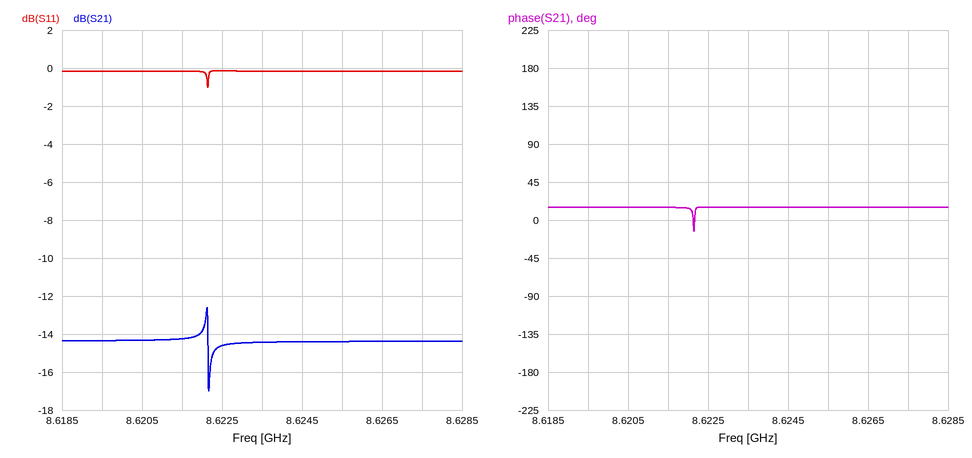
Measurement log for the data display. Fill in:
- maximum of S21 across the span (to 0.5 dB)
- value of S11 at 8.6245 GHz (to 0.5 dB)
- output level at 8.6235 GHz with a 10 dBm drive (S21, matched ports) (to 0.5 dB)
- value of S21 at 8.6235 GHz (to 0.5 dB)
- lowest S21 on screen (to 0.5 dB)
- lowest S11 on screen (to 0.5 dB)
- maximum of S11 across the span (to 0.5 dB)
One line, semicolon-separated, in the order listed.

-12.5 dB; 0.0 dB; -4.5 dBm; -14.5 dB; -17.0 dB; -1.0 dB; 0.0 dB
